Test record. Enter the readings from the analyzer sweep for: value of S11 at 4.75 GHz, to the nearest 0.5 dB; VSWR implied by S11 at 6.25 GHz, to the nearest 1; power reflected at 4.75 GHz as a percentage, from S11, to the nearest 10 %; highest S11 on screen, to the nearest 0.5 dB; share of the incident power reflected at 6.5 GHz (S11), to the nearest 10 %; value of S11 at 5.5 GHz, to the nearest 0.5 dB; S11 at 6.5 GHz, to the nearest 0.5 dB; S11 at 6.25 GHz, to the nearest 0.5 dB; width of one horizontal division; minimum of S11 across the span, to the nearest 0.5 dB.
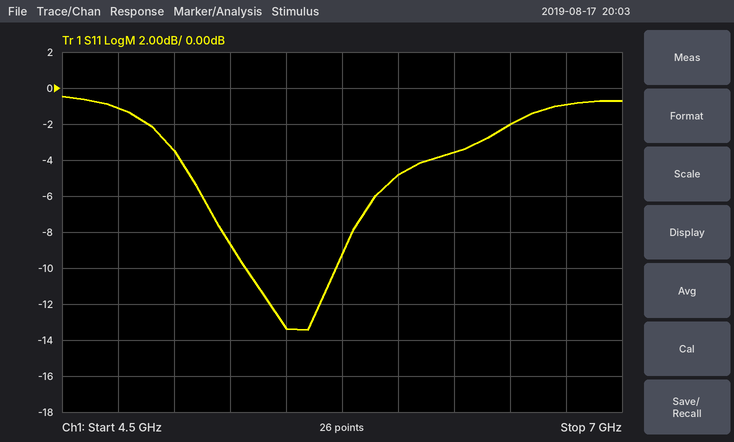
-1.0 dB
5
80 %
-0.5 dB
60 %
-13.5 dB
-2.0 dB
-3.5 dB
250 MHz
-13.5 dB
